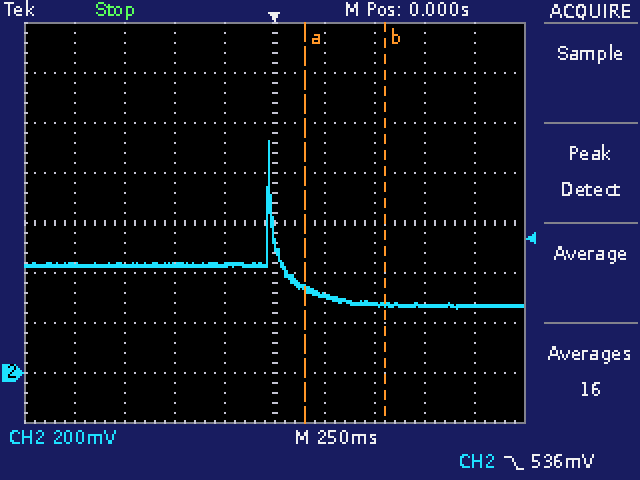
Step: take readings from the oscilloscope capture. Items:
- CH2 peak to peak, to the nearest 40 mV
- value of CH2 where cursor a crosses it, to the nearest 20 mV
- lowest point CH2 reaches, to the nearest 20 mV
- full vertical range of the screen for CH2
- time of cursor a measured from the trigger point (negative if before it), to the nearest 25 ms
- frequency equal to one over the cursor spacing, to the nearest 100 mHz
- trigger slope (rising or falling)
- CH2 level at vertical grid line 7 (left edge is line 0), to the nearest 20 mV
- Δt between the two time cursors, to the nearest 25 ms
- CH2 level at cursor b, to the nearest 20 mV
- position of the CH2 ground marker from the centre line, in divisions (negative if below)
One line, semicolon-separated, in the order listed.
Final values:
680 mV; 340 mV; 260 mV; 1.6 V; +150 ms; 2.5 Hz; falling; 280 mV; 400 ms; 280 mV; -3.0 div
